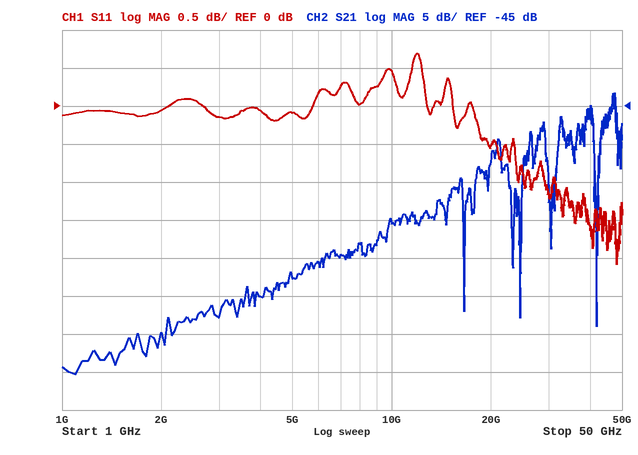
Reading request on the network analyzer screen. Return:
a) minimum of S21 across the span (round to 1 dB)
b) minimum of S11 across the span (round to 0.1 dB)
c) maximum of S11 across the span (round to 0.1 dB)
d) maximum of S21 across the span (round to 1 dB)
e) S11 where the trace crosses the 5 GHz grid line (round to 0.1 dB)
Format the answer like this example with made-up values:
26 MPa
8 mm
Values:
-80 dB
-2.1 dB
0.7 dB
-43 dB
-0.1 dB
